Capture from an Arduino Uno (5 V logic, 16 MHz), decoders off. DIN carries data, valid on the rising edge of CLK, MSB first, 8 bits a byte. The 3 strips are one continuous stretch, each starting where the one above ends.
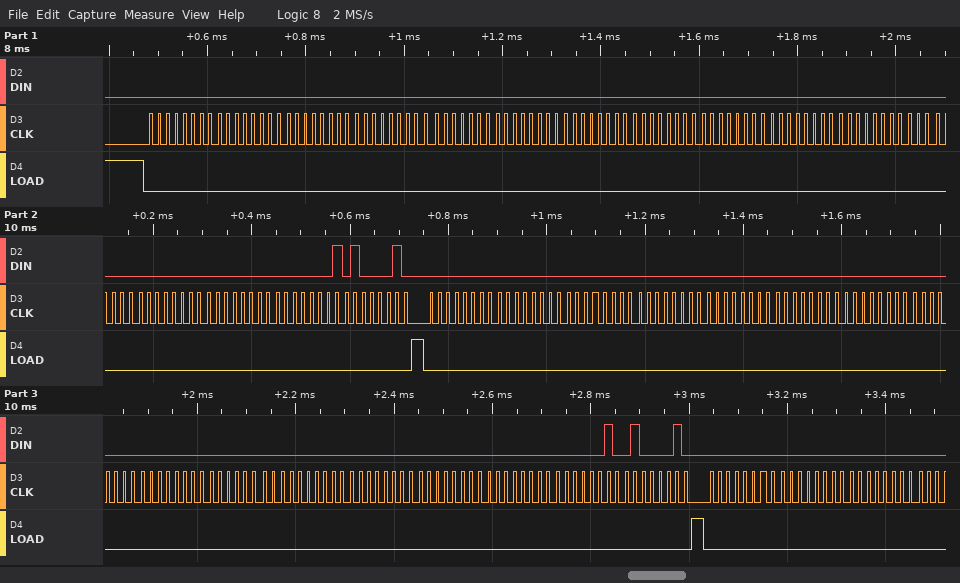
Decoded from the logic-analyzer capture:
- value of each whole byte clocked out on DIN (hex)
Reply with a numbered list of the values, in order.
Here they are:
1. 00 00 00 00 00 00 00 00 00 00 00 00 00 00 01 42 00 00 00 00 00 00 00 00 00 00 00 00 00 00 02 42 00 00 00
